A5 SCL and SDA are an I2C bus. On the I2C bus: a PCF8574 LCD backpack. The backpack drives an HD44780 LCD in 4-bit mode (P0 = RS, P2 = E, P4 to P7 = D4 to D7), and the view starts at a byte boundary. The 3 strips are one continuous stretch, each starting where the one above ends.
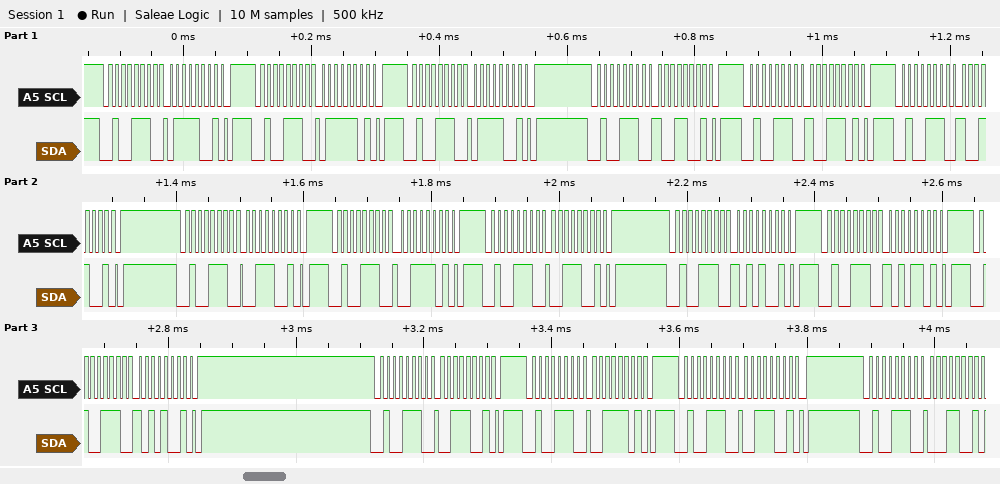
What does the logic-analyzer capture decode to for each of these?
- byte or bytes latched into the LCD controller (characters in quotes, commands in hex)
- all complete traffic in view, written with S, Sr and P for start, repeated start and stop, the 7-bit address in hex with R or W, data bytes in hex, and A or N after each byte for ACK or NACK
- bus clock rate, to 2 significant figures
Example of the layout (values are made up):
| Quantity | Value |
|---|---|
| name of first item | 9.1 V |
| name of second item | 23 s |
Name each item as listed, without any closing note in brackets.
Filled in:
| Quantity | Value |
|---|---|
| byte or bytes latched into the LCD controller | 'y' ':' |
| all complete traffic in view, written with S, Sr and P for start, repeated start and stop, the 7-bit address in hex with R or W, data bytes in hex, and A or N after each byte for ACK or NACK | S 27W A 79 A P S 27W A 7D A P S 27W A 79 A P S 27W A 99 A P S 27W A 9D A P S 27W A 99 A P S 27W A 39 A P S 27W A 3D A P S 27W A 39 A P S 27W A A9 A P S 27W A AD A P S 27W A A9 A P S 27W A 39 A P S 27W A 3D A P S 27W A 39 A P S 27W A 19 A |
| bus clock rate, to 2 significant figures | 100 kHz |
